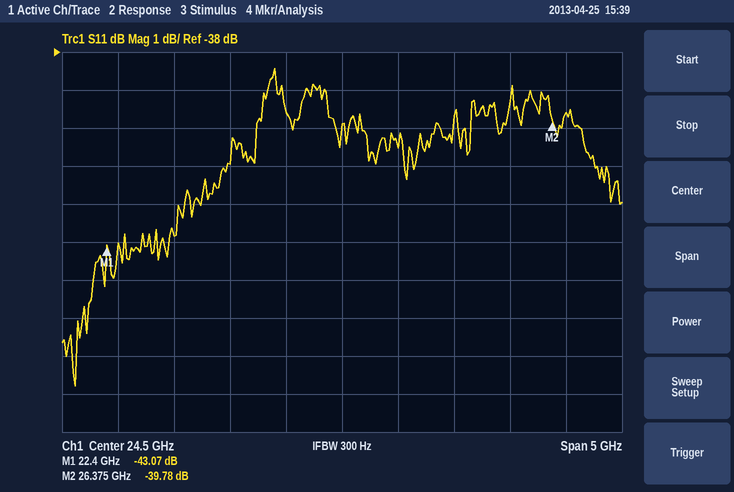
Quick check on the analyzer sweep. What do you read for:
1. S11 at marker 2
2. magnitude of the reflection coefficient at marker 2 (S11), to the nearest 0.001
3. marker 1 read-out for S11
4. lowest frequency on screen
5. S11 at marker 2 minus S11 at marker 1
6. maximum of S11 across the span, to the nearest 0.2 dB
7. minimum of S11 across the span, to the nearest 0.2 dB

-39.78 dB
0.010
-43.07 dB
22 GHz
3.29 dB
-38.4 dB
-46.8 dB
